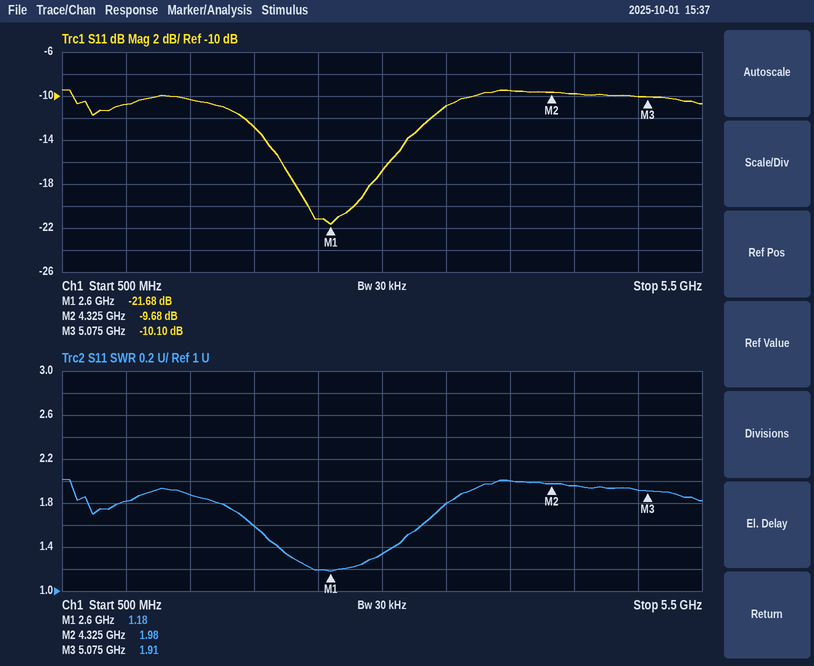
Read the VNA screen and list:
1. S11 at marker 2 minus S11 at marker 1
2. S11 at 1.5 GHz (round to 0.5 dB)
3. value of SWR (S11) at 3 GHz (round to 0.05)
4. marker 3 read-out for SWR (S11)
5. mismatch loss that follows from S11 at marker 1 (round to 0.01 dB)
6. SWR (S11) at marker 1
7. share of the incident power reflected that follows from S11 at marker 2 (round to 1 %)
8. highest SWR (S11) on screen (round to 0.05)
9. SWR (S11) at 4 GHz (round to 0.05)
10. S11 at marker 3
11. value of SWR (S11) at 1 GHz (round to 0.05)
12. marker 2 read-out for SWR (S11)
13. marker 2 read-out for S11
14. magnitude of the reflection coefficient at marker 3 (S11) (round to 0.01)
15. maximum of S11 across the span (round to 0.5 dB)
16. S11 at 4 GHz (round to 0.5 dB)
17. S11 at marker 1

12.00 dB
-10.5 dB
1.35
1.91
0.03 dB
1.18
11 %
2.00
2.00
-10.10 dB
1.80
1.98
-9.68 dB
0.31
-9.5 dB
-9.5 dB
-21.68 dB
